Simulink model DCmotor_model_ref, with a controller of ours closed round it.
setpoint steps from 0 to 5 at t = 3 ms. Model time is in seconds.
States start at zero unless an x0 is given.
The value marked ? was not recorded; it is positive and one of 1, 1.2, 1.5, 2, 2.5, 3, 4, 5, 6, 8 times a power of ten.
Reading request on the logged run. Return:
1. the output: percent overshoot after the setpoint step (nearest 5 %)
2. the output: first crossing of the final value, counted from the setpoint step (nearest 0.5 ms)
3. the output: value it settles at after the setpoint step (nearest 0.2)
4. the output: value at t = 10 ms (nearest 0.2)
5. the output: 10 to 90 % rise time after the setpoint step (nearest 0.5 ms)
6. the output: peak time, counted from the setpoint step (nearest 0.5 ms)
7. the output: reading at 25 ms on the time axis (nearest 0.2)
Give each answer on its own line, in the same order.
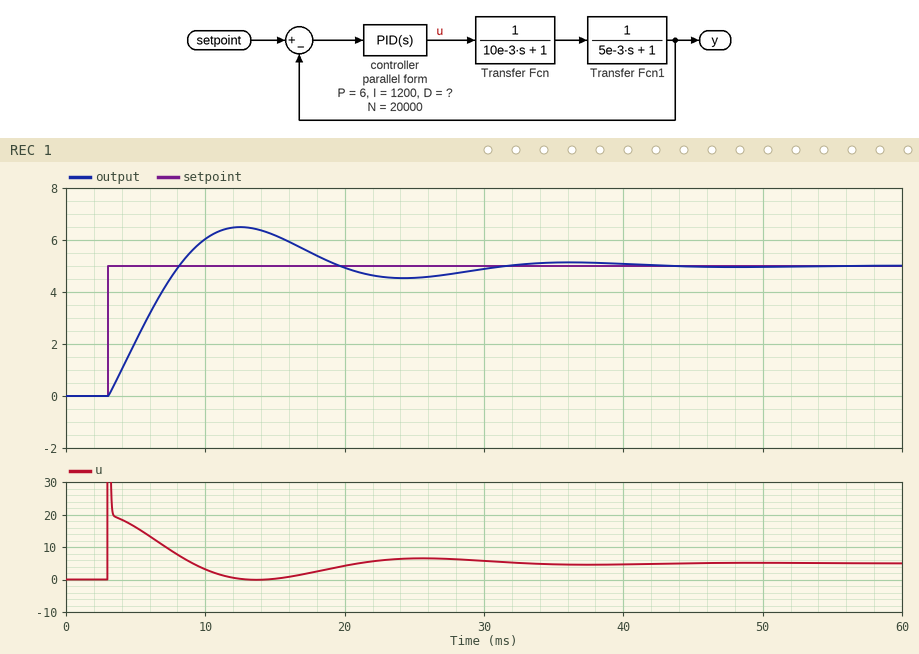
30 %
5.0 ms
5.0
6.0
4.0 ms
9.5 ms
4.6
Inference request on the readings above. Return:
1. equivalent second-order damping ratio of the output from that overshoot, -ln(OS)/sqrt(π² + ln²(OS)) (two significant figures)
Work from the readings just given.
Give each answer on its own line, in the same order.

0.36
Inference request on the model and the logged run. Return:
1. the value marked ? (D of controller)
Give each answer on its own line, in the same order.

0.01
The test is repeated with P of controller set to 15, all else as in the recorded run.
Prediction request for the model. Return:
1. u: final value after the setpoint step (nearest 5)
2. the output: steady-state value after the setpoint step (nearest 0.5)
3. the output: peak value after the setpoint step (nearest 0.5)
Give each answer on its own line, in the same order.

5
5.0
6.5
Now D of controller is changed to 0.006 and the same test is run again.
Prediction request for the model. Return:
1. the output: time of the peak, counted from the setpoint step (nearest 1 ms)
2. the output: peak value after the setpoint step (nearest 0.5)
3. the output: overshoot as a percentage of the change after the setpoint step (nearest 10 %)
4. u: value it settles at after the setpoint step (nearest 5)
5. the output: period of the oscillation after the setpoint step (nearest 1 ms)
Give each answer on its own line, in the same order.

9 ms
7.0
40 %
5
21 ms
